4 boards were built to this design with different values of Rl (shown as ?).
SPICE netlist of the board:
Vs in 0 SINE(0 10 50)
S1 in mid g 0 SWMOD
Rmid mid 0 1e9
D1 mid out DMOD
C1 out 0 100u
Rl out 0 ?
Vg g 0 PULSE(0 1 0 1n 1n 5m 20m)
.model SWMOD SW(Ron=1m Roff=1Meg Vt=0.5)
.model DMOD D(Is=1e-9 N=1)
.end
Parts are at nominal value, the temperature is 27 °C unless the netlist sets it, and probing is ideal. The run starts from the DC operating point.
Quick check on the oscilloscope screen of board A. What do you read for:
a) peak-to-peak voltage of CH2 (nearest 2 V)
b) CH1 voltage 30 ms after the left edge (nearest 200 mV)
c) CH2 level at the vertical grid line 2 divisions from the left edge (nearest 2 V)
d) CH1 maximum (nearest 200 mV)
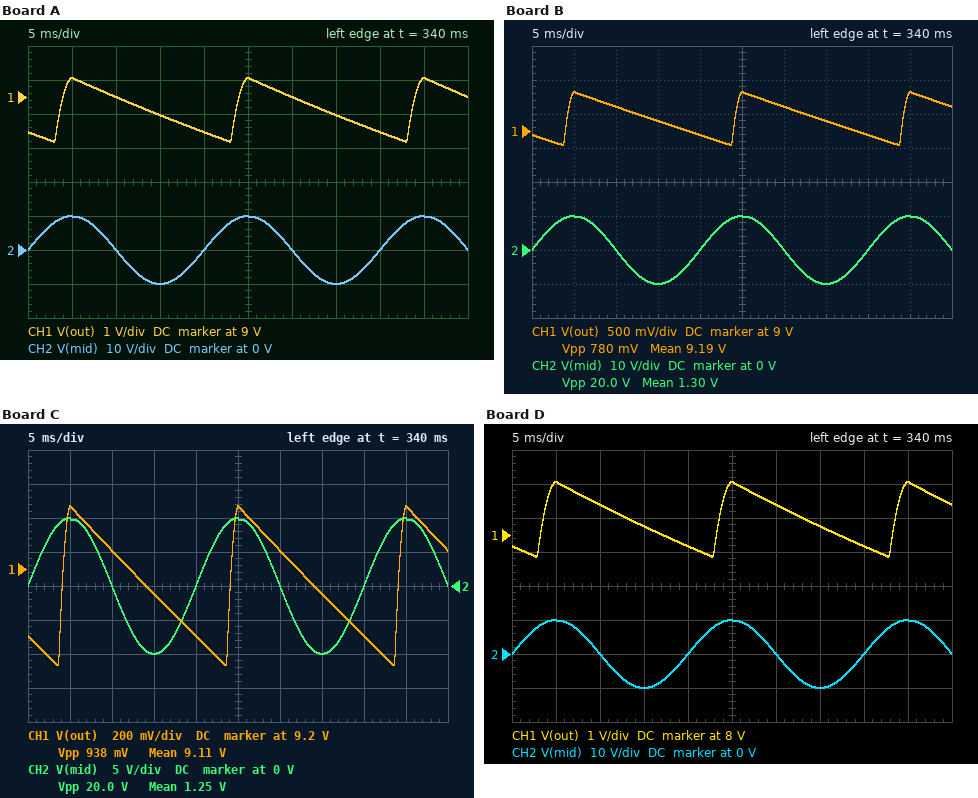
20 V
9.0 V
0 V
9.6 V
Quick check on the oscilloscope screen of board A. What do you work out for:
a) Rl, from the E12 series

820 Ω
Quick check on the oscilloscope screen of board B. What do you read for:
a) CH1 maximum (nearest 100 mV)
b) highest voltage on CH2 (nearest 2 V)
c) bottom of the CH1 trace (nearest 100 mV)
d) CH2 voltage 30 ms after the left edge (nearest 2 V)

9.6 V
10 V
8.8 V
0 V
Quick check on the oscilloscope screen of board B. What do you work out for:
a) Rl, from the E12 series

2.2 kΩ
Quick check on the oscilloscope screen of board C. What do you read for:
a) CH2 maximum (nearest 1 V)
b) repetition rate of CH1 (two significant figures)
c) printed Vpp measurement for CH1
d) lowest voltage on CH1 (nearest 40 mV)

10 V
50 Hz
938 mV
8.64 V
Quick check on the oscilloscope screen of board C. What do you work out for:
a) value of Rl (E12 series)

1.8 kΩ
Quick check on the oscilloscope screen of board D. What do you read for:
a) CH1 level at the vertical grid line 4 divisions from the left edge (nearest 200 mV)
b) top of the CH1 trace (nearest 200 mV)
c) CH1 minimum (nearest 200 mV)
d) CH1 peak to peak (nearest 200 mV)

7.6 V
9.6 V
7.4 V
2.2 V
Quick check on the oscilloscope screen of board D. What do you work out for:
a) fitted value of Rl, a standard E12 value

680 Ω
